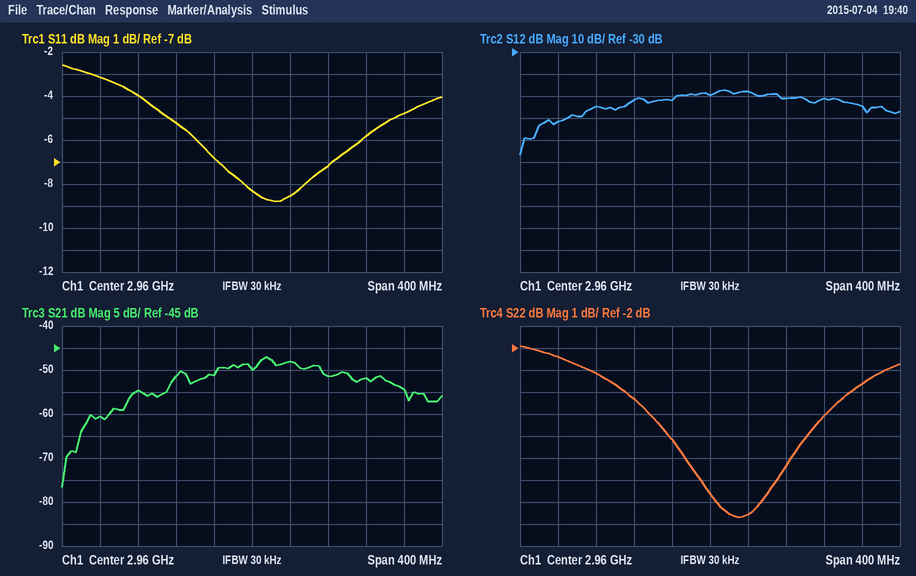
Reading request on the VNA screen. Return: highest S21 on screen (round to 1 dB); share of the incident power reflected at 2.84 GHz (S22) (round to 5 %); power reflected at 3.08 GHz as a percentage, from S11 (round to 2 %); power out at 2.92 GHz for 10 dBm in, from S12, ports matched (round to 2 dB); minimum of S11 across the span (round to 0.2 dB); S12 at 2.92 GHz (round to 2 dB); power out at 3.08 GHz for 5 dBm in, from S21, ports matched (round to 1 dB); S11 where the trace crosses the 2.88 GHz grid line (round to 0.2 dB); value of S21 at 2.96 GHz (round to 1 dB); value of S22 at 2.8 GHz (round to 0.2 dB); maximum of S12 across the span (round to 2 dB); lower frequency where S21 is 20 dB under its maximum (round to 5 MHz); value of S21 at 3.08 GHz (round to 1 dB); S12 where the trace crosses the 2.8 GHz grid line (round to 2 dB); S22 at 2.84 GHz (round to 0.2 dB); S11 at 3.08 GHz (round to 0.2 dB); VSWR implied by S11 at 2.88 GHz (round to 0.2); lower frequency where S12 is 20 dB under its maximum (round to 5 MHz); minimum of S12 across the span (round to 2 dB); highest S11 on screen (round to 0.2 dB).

-47 dB
50 %
26 %
-42 dBm
-8.8 dB
-52 dB
-47 dBm
-5.2 dB
-50 dB
-2.4 dB
-48 dB
2.775 GHz
-52 dB
-62 dB
-3.2 dB
-5.8 dB
3.4
2.775 GHz
-76 dB
-2.6 dB
